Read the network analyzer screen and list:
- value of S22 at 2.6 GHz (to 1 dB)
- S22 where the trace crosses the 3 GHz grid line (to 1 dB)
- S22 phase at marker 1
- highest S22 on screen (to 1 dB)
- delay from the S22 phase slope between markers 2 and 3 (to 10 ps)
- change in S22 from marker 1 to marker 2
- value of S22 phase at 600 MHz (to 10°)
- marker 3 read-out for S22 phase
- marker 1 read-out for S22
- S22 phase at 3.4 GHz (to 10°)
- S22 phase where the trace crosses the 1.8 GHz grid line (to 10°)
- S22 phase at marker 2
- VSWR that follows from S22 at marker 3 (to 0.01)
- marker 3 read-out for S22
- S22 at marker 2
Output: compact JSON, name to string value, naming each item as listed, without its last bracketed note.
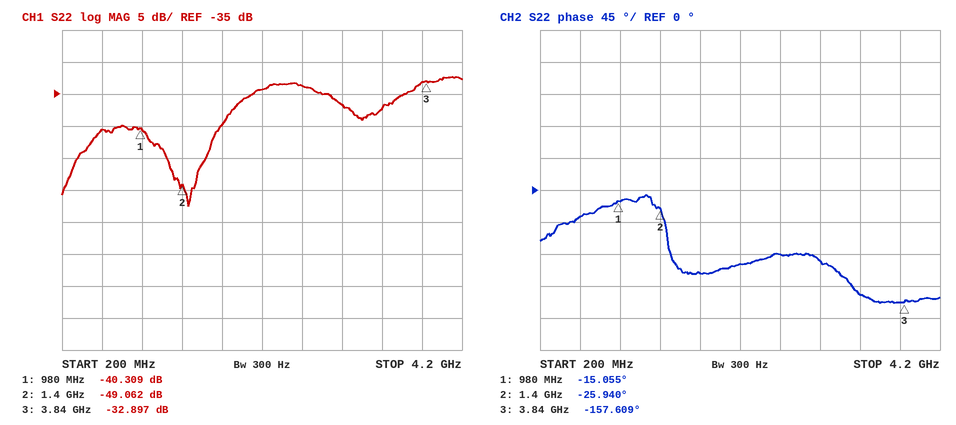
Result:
{"value of S22 at 2.6 GHz": "-34 dB", "S22 where the trace crosses the 3 GHz grid line": "-37 dB", "S22 phase at marker 1": "-15.055°", "highest S22 on screen": "-32 dB", "delay from the S22 phase slope between markers 2 and 3": "150 ps", "change in S22 from marker 1 to marker 2": "-8.753 dB", "value of S22 phase at 600 MHz": "-40°", "marker 3 read-out for S22 phase": "-157.609°", "marker 1 read-out for S22": "-40.309 dB", "S22 phase at 3.4 GHz": "-150°", "S22 phase where the trace crosses the 1.8 GHz grid line": "-120°", "S22 phase at marker 2": "-25.940°", "VSWR that follows from S22 at marker 3": "1.05", "marker 3 read-out for S22": "-32.897 dB", "S22 at marker 2": "-49.062 dB"}
